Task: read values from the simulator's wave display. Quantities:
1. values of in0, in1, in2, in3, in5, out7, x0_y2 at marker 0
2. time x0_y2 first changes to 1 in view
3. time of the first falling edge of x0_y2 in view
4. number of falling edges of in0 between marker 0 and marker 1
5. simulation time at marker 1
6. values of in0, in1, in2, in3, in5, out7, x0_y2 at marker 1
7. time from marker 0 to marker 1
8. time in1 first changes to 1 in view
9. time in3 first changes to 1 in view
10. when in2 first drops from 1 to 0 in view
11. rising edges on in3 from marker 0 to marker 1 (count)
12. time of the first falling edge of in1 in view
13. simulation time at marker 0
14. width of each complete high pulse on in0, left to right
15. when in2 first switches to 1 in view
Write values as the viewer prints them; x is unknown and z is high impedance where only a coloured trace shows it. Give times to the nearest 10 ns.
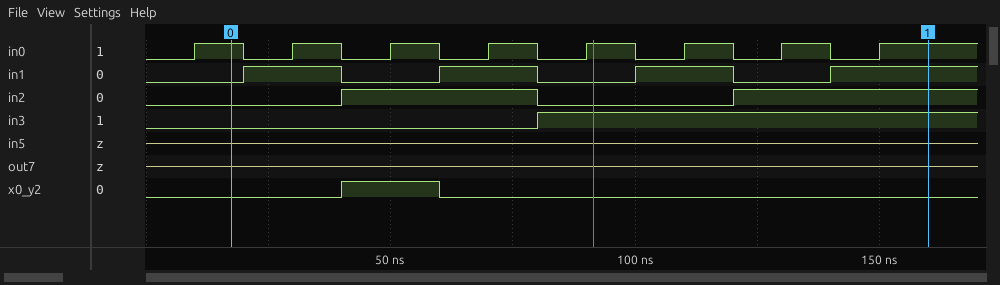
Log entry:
in0=1, in1=0, in2=0, in3=0, in5=z, out7=z, x0_y2=0
40 ns
60 ns
7
160 ns
in0=1, in1=1, in2=1, in3=1, in5=z, out7=z, x0_y2=0
140 ns
20 ns
80 ns
80 ns
1
40 ns
20 ns
10 ns, 10 ns, 10 ns, 10 ns, 10 ns, 10 ns, 10 ns
40 ns
